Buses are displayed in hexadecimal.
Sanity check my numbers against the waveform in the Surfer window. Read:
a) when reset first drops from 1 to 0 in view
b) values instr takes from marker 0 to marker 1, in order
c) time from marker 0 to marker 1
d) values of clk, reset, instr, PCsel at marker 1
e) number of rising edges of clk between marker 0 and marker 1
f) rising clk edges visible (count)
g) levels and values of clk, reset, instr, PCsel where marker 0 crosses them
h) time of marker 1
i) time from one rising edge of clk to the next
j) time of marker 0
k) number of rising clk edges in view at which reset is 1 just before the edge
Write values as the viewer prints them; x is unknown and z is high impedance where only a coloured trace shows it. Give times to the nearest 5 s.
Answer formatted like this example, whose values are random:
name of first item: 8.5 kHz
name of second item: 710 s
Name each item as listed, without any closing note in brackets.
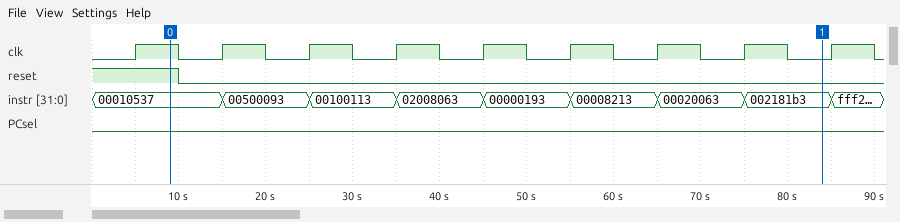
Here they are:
when reset first drops from 1 to 0 in view: 10 s
values instr takes from marker 0 to marker 1, in order: 00010537, 00500093, 00100113, 02008063, 00000193, 00008213, 00020063, 002181b3
time from marker 0 to marker 1: 75 s
values of clk, reset, instr, PCsel at marker 1: clk=0, reset=0, instr=002181b3, PCsel=0
number of rising edges of clk between marker 0 and marker 1: 7
rising clk edges visible: 9
levels and values of clk, reset, instr, PCsel where marker 0 crosses them: clk=1, reset=1, instr=00010537, PCsel=0
time of marker 1: 85 s
time from one rising edge of clk to the next: 10 s
time of marker 0: 10 s
number of rising clk edges in view at which reset is 1 just before the edge: 1
